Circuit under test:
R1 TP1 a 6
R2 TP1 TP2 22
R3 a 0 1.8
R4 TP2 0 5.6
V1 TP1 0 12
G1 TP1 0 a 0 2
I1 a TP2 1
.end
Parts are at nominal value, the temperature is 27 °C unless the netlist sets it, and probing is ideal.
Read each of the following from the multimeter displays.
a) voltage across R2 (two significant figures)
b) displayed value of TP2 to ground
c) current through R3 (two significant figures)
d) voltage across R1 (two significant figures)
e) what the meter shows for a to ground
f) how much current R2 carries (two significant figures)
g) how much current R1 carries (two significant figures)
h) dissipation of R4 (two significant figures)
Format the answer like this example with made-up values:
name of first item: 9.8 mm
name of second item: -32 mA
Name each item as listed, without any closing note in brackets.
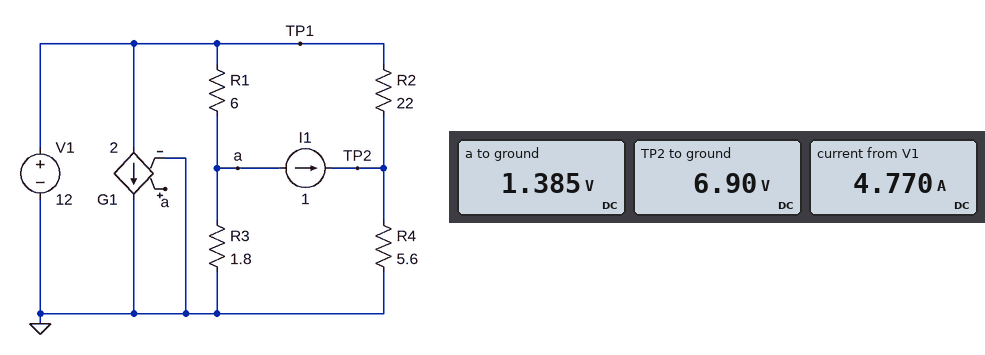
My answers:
voltage across R2: 5.1 V
displayed value of TP2 to ground: 6.90 V
current through R3: 770 mA
voltage across R1: 11 V
what the meter shows for a to ground: 1.385 V
how much current R2 carries: 230 mA
how much current R1 carries: 1.8 A
dissipation of R4: 8.5 W
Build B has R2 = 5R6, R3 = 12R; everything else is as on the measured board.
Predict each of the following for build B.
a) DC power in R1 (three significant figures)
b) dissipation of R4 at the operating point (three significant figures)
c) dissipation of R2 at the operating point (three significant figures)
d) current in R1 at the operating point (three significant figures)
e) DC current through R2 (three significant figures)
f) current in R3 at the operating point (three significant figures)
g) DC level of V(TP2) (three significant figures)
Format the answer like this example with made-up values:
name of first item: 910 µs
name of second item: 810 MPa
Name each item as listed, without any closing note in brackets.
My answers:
DC power in R1: 10.7 W
dissipation of R4 at the operating point: 13.8 W
dissipation of R2 at the operating point: 1.83 W
current in R1 at the operating point: 1.33 A
DC current through R2: 571 mA
current in R3 at the operating point: 333 mA
DC level of V(TP2): 8.80 V
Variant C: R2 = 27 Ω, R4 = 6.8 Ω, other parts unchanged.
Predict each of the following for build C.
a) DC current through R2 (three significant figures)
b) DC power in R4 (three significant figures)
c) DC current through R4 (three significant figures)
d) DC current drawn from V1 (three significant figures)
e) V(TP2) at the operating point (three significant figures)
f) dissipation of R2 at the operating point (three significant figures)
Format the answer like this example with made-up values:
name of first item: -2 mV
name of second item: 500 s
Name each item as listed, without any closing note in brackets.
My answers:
DC current through R2: 154 mA
DC power in R4: 9.05 W
DC current through R4: 1.15 A
DC current drawn from V1: 4.69 A
V(TP2) at the operating point: 7.85 V
dissipation of R2 at the operating point: 639 mW
